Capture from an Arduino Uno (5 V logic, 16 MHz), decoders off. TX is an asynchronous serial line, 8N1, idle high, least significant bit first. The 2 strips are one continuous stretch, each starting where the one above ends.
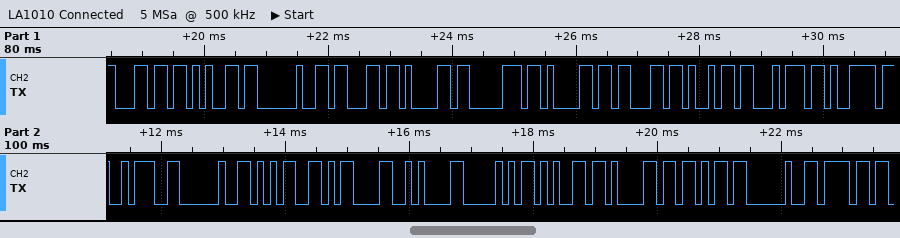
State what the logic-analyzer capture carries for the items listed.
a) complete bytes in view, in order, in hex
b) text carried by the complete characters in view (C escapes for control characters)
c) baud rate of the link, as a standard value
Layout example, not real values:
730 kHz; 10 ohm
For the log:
6C 65 20 63 61 70 61 63 69 74 79 3A 20 35 0D 0A 50 65 61 6B 20 6F; "le capacity: 5\r\nPeak o"; 9600 baud
